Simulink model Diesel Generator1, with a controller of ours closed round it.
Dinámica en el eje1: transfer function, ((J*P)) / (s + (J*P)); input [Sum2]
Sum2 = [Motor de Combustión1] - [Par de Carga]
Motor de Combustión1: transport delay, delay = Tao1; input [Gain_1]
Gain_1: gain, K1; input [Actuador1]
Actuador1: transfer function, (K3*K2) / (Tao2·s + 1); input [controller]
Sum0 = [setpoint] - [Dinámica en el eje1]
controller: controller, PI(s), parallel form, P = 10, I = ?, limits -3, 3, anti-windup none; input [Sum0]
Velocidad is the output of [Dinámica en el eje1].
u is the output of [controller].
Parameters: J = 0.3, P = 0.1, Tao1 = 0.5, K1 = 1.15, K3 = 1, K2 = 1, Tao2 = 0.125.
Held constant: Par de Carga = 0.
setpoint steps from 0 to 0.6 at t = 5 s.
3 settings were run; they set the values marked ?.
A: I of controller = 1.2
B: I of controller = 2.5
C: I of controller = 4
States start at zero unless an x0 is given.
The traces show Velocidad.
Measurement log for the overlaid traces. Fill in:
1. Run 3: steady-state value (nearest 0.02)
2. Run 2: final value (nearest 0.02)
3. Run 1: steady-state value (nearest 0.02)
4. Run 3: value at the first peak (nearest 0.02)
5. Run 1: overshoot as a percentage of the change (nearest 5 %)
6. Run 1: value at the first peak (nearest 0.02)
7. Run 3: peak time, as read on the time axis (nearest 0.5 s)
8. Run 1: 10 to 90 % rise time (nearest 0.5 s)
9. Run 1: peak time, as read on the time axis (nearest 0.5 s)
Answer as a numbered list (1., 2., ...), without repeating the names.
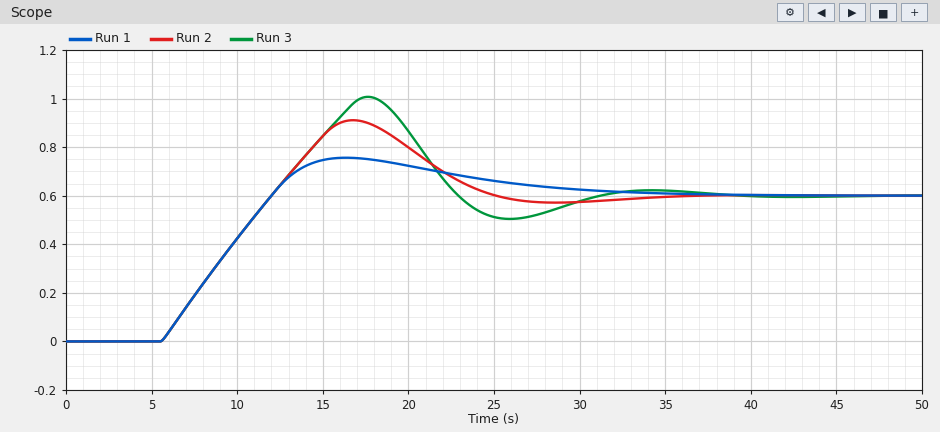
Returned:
1. 0.60
2. 0.60
3. 0.60
4. 1.00
5. 25 %
6. 0.76
7. 17.5 s
8. 5.0 s
9. 16.5 s
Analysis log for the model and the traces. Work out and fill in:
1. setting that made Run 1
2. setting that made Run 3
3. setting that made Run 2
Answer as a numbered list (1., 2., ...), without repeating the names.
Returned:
1. A
2. C
3. B
